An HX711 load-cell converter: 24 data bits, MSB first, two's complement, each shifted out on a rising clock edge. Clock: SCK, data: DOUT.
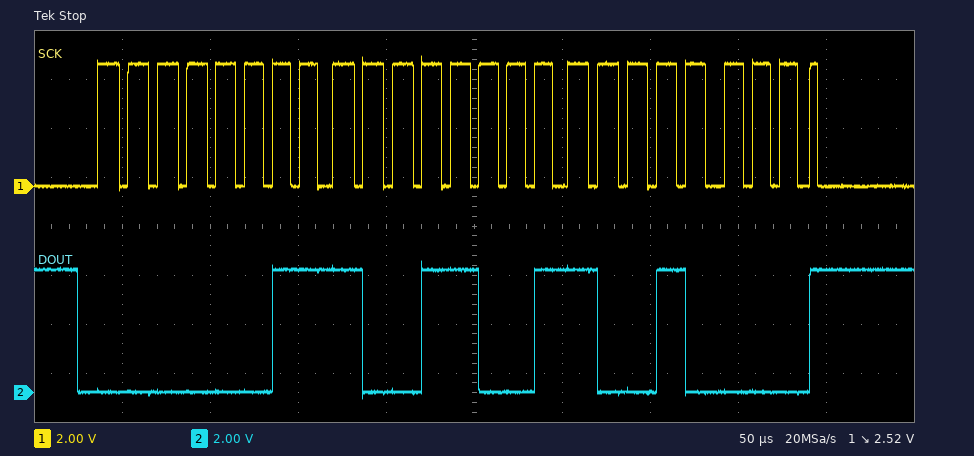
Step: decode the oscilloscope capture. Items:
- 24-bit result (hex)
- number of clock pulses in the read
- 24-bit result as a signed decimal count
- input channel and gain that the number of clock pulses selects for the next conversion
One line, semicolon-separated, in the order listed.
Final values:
0x039990; 25; 235920; channel A, gain 128
